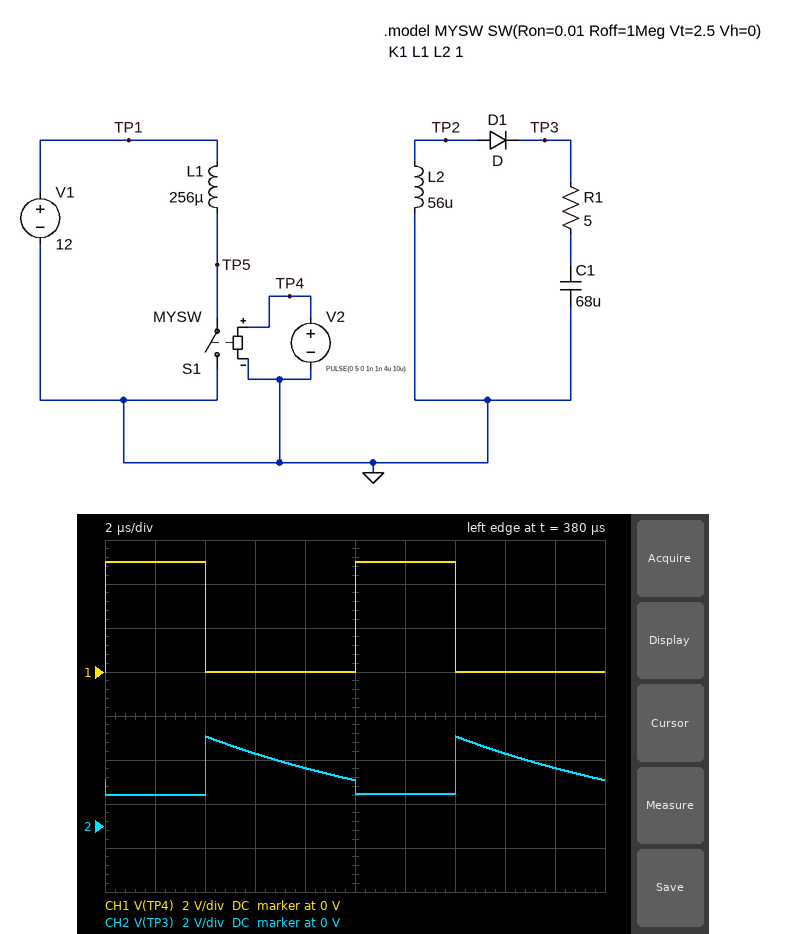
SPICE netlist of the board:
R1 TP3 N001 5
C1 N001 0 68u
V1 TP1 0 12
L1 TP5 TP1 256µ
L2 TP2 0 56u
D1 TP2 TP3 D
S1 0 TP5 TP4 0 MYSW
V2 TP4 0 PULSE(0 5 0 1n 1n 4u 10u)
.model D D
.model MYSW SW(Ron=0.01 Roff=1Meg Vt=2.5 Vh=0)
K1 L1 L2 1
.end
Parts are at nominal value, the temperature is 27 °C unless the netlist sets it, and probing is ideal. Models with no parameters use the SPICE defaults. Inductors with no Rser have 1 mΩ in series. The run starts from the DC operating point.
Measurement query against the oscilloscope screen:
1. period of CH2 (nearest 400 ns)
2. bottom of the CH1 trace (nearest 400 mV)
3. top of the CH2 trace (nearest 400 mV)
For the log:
10.0 µs
0 V
4.0 V
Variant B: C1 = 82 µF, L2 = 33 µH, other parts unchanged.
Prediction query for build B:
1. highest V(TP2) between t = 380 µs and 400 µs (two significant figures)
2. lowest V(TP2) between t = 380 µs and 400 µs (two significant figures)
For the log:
4.4 V
-4.3 V
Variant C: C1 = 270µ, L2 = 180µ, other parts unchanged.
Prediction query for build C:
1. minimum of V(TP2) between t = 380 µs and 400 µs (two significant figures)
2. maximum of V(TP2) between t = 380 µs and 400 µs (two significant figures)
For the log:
-10 V
7.4 V
